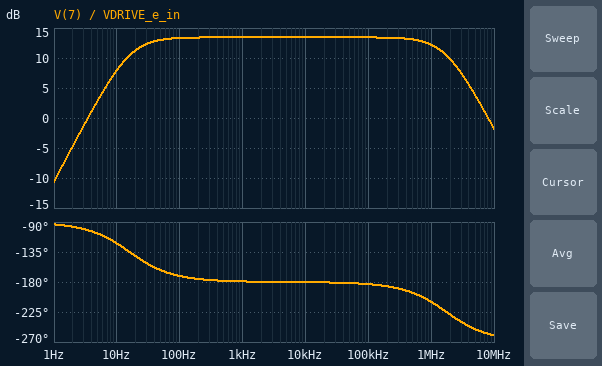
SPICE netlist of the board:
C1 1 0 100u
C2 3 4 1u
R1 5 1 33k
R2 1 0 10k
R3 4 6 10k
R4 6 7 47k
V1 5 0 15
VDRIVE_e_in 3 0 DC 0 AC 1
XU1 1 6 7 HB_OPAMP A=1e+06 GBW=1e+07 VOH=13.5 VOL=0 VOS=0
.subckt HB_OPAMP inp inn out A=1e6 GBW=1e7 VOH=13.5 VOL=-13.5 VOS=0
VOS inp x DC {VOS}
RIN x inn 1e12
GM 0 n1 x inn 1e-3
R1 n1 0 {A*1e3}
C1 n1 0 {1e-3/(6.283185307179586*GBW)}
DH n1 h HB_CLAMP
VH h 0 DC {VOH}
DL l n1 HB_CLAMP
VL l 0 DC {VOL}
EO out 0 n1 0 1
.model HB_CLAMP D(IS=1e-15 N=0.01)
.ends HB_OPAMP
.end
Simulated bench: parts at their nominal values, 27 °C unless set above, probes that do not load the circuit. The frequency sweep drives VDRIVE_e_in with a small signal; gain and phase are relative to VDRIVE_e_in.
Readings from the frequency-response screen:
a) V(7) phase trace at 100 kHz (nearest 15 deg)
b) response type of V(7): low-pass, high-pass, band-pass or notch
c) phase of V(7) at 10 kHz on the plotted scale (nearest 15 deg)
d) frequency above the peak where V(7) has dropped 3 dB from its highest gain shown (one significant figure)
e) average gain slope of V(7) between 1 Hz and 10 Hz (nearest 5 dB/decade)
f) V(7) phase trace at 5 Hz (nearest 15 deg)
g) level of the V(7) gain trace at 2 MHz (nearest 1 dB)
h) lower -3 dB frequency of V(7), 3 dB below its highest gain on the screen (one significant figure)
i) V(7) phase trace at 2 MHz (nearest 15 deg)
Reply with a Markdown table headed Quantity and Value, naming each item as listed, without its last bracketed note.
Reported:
| Quantity | Value |
|---|---|
| V(7) phase trace at 100 kHz | -180 deg |
| response type of V(7): low-pass, high-pass, band-pass or notch | band-pass |
| phase of V(7) at 10 kHz on the plotted scale | -180 deg |
| frequency above the peak where V(7) has dropped 3 dB from its highest gain shown | 2 MHz |
| average gain slope of V(7) between 1 Hz and 10 Hz | 20 dB/decade |
| V(7) phase trace at 5 Hz | -105 deg |
| level of the V(7) gain trace at 2 MHz | 10 dB |
| lower -3 dB frequency of V(7), 3 dB below its highest gain on the screen | 20 Hz |
| V(7) phase trace at 2 MHz | -225 deg |
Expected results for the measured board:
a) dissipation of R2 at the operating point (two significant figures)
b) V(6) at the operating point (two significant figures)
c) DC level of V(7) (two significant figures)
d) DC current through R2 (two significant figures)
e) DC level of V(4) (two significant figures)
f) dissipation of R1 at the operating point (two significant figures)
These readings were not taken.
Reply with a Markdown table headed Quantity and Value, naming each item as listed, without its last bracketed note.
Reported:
| Quantity | Value |
|---|---|
| dissipation of R2 at the operating point | 1.2 mW |
| V(6) at the operating point | 3.5 V |
| DC level of V(7) | 3.5 V |
| DC current through R2 | 350 µA |
| DC level of V(4) | 3.5 V |
| dissipation of R1 at the operating point | 4.0 mW |
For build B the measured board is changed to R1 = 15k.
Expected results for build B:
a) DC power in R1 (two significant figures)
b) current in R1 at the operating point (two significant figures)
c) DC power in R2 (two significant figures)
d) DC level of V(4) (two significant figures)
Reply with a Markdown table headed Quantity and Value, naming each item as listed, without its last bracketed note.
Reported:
| Quantity | Value |
|---|---|
| DC power in R1 | 5.4 mW |
| current in R1 at the operating point | 600 µA |
| DC power in R2 | 3.6 mW |
| DC level of V(4) | 6.0 V |
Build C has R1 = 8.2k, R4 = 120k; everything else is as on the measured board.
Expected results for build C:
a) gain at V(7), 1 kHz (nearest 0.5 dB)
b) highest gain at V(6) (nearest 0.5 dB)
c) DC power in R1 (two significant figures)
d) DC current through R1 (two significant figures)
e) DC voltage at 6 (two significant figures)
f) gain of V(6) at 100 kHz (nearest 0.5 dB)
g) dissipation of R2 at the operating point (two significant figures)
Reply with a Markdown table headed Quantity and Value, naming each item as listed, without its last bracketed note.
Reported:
| Quantity | Value |
|---|---|
| gain at V(7), 1 kHz | 21.5 dB |
| highest gain at V(6) | -0.5 dB |
| DC power in R1 | 5.6 mW |
| DC current through R1 | 820 µA |
| DC voltage at 6 | 8.2 V |
| gain of V(6) at 100 kHz | -18.5 dB |
| dissipation of R2 at the operating point | 6.8 mW |
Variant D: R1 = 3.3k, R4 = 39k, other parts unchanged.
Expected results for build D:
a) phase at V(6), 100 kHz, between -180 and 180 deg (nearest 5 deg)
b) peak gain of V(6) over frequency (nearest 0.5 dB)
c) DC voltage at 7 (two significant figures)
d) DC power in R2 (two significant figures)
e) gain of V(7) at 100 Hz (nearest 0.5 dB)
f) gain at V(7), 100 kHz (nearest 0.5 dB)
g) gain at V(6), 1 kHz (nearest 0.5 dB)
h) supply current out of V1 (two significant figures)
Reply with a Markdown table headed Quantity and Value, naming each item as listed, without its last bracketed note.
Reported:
| Quantity | Value |
|---|---|
| phase at V(6), 100 kHz, between -180 and 180 deg | 85 deg |
| peak gain of V(6) over frequency | -2.0 dB |
| DC voltage at 7 | 11 V |
| DC power in R2 | 13 mW |
| gain of V(7) at 100 Hz | 11.5 dB |
| gain at V(7), 100 kHz | 12.0 dB |
| gain at V(6), 1 kHz | -68.0 dB |
| supply current out of V1 | 1.1 mA |
